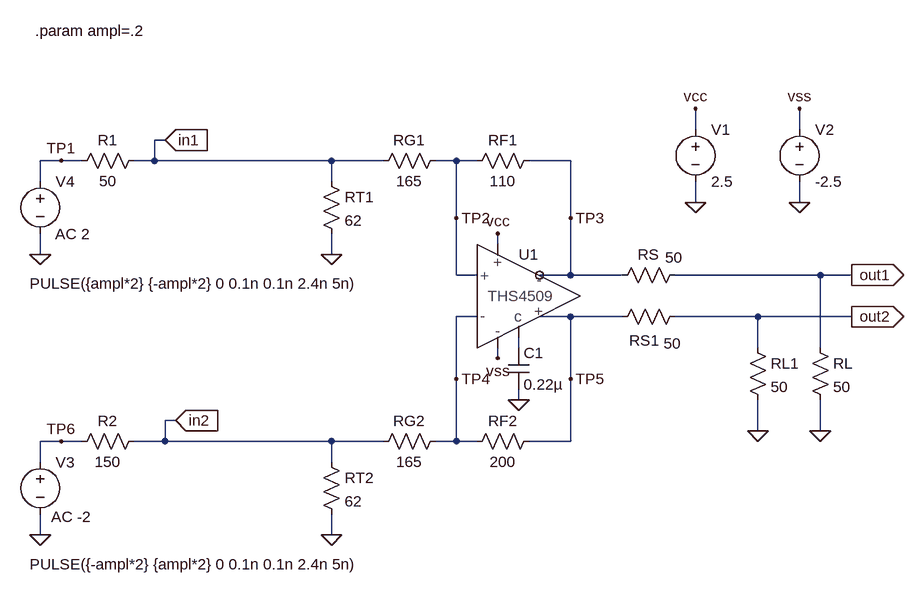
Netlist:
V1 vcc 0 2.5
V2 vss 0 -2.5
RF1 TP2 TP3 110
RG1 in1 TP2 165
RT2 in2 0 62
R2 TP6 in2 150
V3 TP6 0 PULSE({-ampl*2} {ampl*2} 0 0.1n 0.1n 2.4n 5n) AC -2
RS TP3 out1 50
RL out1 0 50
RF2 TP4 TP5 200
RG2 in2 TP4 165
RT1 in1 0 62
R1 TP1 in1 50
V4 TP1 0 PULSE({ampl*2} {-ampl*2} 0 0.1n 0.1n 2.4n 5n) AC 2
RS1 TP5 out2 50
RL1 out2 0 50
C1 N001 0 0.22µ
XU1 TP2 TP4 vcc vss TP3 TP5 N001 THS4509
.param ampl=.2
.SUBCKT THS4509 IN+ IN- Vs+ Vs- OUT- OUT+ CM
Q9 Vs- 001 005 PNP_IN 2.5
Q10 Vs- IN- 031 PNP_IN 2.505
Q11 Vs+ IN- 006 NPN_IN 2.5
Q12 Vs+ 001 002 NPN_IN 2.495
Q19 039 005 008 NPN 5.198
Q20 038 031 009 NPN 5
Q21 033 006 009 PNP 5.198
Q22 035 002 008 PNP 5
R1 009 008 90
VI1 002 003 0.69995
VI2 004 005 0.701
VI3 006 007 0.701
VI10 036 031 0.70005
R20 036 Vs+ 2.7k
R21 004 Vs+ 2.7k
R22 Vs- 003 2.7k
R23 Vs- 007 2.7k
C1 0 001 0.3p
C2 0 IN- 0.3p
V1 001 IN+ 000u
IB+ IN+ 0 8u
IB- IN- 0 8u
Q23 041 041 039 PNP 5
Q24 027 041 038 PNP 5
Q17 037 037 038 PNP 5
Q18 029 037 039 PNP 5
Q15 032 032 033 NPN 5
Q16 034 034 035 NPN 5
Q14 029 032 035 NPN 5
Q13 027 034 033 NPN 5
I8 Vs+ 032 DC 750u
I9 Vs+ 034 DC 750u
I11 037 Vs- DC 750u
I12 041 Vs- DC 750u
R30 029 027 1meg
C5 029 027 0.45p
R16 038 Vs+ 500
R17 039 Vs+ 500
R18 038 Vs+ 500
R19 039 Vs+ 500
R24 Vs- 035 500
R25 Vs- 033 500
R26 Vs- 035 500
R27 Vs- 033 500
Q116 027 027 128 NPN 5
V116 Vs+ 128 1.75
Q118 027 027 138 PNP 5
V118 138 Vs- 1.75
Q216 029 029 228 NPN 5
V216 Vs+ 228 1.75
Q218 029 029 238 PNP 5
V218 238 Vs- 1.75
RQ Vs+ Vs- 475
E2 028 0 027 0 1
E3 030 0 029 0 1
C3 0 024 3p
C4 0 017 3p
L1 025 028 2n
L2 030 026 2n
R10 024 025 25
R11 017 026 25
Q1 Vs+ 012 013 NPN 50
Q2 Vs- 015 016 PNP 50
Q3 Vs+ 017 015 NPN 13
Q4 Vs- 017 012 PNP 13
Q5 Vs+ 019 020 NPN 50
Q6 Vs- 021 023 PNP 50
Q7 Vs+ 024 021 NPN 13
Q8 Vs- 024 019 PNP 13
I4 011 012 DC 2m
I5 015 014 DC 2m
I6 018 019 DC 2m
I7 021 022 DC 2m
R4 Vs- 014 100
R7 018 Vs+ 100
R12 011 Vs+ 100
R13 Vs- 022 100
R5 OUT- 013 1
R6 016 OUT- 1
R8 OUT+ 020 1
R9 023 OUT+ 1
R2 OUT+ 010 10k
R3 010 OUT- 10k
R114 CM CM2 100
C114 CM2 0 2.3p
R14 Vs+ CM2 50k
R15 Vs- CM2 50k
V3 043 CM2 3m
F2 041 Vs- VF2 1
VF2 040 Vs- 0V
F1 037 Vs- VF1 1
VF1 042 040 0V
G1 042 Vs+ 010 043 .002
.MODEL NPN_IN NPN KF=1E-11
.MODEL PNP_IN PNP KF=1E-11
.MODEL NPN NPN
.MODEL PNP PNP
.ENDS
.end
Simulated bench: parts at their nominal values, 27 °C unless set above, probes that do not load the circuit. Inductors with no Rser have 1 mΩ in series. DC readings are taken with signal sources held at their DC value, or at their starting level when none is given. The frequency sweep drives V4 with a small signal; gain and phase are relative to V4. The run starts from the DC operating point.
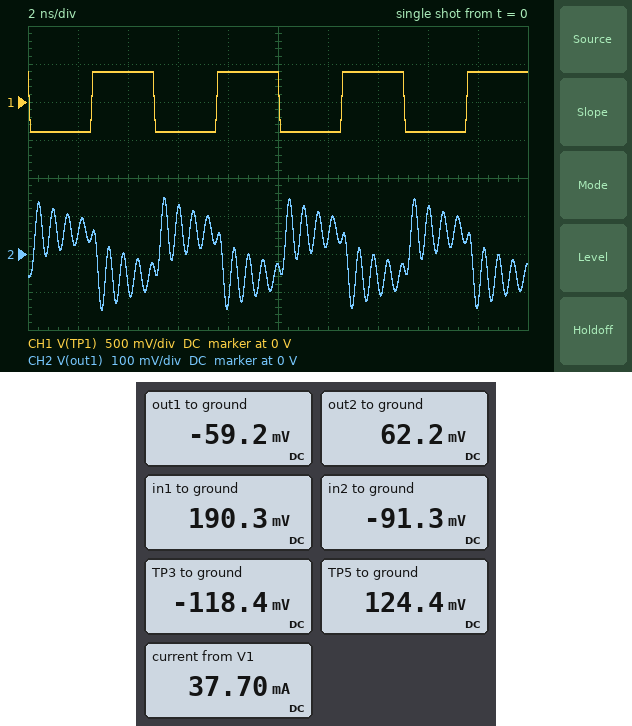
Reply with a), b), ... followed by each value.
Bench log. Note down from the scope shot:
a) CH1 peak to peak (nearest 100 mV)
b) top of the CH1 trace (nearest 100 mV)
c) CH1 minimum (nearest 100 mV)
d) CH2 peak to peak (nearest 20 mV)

a) 800 mV
b) 400 mV
c) -400 mV
d) 300 mV
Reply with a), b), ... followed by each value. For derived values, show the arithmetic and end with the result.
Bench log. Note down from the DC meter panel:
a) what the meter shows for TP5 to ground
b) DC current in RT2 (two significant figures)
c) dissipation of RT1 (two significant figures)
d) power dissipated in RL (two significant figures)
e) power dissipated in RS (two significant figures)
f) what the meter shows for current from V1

a) 124.4 mV
b) (0 V - (-91.3 mV)) / 62 Ω = 1.5 mA
c) (190.3 mV)^2 / 62 Ω = 580 µW
d) (0 V - (-59.2 mV))^2 / 50 Ω = 70 µW
e) (-59.2 mV - (-118.4 mV))^2 / 50 Ω = 70 µW
f) 37.70 mA
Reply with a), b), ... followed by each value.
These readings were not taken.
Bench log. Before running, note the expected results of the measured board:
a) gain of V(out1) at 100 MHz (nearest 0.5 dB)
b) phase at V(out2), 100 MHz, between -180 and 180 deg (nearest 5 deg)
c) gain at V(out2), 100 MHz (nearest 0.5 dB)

a) -13.5 dB
b) -5 deg
c) -13.5 dB
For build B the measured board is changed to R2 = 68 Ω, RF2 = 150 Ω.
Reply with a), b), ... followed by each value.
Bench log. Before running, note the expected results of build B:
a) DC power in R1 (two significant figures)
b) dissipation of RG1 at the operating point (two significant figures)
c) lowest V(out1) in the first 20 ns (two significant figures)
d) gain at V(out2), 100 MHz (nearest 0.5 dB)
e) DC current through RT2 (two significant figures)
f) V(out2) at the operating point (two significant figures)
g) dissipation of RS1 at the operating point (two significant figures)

a) 890 µW
b) 230 µW
c) -490 mV
d) -12.0 dB
e) 2.6 mA
f) 70 mV
g) 97 µW
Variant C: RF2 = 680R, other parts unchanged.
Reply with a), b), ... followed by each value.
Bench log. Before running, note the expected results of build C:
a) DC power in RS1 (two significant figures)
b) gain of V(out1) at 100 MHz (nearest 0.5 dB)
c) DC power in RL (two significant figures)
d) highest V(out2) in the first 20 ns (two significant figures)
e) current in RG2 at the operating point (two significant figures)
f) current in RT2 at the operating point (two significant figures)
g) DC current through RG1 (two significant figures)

a) 200 µW
b) -8.5 dB
c) 190 µW
d) 180 mV
e) 350 µA
f) 1.6 mA
g) 1.4 mA
